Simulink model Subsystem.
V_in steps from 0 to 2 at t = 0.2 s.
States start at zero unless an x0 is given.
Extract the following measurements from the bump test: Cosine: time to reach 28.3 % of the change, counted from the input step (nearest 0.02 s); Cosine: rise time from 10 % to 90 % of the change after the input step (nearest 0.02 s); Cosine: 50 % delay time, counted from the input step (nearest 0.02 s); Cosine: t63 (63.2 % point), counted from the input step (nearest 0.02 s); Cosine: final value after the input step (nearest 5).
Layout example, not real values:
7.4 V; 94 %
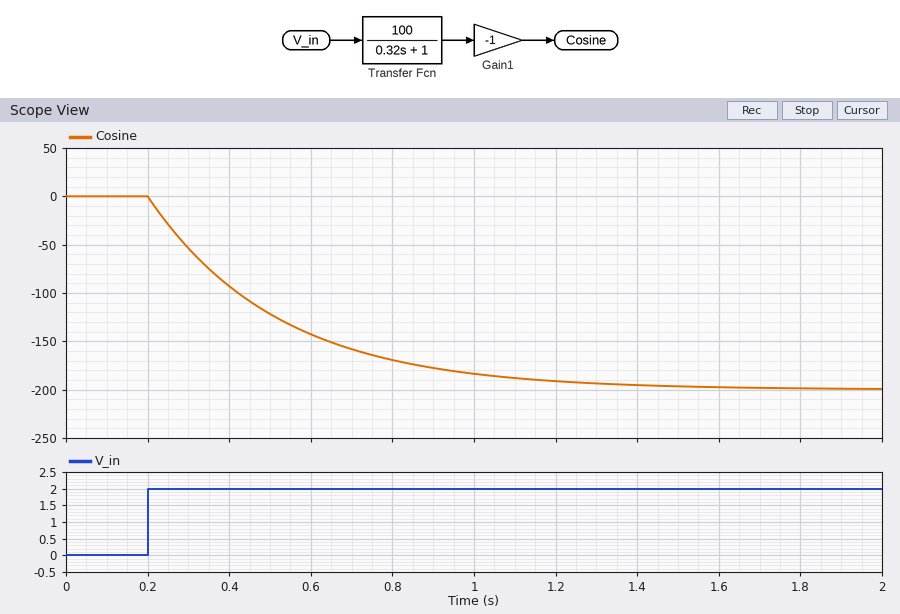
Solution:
0.10 s; 0.70 s; 0.22 s; 0.32 s; -200
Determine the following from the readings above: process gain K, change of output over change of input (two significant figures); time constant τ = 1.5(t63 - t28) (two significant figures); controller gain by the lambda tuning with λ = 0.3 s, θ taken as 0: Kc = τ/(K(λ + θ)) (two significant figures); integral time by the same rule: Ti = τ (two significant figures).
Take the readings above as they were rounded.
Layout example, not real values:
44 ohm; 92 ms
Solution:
-100; 0.33 s; -0.011; 0.33 s
